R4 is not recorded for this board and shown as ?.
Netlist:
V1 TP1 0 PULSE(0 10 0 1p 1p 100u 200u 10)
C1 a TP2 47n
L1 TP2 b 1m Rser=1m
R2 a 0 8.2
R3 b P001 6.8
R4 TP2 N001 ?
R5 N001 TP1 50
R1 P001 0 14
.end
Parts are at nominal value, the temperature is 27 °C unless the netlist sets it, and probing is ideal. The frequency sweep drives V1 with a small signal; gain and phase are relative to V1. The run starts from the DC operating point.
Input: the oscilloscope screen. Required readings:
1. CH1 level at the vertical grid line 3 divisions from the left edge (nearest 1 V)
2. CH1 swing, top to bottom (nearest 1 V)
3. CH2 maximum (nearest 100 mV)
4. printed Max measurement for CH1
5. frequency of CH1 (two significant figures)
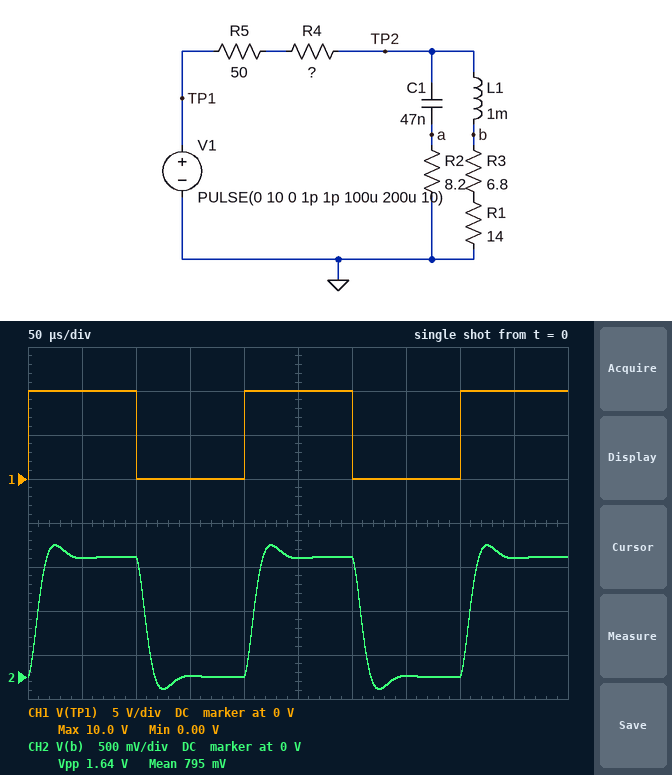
0 V
10 V
1.5 V
10.0 V
5.0 kHz
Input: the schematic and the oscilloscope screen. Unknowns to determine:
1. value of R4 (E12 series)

82 Ω
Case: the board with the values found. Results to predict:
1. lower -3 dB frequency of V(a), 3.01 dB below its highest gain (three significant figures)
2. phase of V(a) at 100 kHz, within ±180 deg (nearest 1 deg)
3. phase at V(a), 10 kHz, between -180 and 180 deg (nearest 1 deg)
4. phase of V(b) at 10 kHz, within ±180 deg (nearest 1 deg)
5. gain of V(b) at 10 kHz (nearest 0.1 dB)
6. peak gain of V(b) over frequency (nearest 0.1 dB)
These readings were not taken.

21.5 kHz
15 deg
131 deg
-29 deg
-17.0 dB
-16.9 dB
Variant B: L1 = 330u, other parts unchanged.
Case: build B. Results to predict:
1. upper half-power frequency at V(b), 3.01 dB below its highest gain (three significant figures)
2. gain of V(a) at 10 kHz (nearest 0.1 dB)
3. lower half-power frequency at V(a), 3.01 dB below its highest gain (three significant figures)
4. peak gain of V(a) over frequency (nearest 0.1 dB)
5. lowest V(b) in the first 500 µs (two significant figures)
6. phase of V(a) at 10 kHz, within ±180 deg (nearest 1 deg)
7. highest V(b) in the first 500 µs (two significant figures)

50.0 kHz
-46.4 dB
35.2 kHz
-22.6 dB
-280 mV
122 deg
1.6 V
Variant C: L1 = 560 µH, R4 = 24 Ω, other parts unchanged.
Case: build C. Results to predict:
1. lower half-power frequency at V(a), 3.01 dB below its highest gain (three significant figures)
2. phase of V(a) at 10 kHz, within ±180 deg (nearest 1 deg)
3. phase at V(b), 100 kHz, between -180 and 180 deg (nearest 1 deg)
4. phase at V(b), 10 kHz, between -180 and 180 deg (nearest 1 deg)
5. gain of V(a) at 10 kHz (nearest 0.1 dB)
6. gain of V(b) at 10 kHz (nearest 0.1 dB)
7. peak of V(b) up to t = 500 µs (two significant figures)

34.3 kHz
123 deg
-137 deg
-25 deg
-39.7 dB
-13.3 dB
2.3 V
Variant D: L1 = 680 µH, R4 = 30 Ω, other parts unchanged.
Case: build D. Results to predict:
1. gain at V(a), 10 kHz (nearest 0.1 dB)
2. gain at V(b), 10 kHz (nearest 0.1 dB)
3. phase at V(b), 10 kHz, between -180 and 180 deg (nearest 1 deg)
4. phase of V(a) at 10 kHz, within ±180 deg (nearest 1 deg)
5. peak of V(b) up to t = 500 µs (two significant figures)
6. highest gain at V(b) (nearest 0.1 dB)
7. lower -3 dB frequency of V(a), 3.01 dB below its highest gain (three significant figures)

-39.0 dB
-13.9 dB
-28 deg
125 deg
2.1 V
-13.7 dB
31.5 kHz
